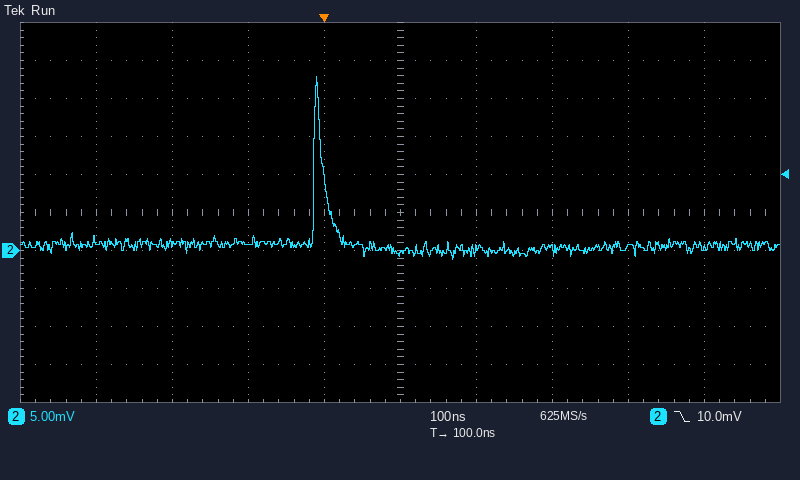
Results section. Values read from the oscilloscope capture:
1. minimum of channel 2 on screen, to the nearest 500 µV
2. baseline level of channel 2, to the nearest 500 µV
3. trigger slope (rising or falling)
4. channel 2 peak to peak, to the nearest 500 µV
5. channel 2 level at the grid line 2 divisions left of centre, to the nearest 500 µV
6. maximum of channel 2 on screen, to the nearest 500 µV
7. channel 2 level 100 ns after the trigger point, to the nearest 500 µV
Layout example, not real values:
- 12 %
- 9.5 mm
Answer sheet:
- -1.0 mV
- 500 µV
- falling
- 24.0 mV
- 1.0 mV
- 23.0 mV
- -500 µV
